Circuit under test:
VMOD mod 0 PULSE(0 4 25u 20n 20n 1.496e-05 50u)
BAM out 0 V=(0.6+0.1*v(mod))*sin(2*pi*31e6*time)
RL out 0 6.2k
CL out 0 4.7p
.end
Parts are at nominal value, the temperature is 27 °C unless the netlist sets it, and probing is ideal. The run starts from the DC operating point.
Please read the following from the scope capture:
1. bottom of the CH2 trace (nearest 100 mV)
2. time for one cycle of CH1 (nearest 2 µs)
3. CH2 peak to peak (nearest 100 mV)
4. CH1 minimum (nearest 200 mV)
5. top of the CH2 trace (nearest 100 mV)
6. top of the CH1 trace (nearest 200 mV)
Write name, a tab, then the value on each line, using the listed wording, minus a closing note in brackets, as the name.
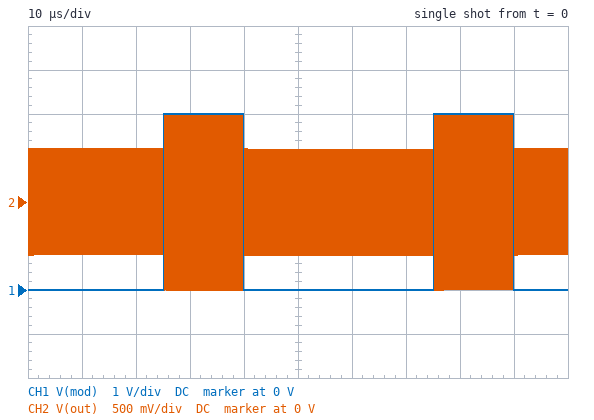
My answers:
bottom of the CH2 trace	-1.0 V
time for one cycle of CH1	50 µs
CH2 peak to peak	2.0 V
CH1 minimum	0 V
top of the CH2 trace	1.0 V
top of the CH1 trace	4.0 V
